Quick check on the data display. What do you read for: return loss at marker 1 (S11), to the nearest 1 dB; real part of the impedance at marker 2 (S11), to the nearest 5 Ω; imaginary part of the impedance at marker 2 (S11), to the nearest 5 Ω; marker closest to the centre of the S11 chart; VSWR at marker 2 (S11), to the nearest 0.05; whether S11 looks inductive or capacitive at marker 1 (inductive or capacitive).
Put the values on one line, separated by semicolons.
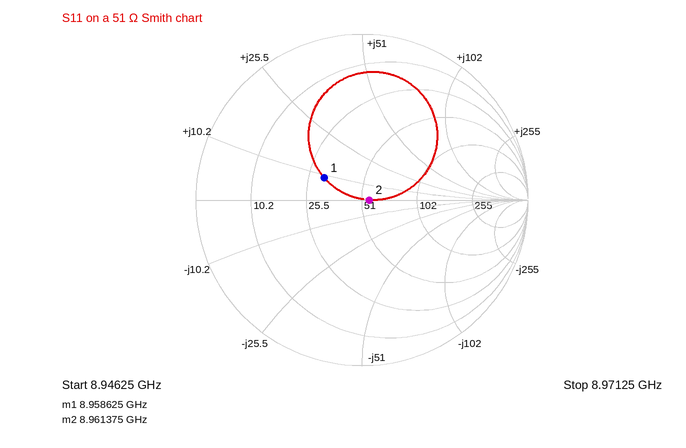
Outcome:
12 dB; 55 Ω; 0 Ω; marker 2; 1.10; inductive
